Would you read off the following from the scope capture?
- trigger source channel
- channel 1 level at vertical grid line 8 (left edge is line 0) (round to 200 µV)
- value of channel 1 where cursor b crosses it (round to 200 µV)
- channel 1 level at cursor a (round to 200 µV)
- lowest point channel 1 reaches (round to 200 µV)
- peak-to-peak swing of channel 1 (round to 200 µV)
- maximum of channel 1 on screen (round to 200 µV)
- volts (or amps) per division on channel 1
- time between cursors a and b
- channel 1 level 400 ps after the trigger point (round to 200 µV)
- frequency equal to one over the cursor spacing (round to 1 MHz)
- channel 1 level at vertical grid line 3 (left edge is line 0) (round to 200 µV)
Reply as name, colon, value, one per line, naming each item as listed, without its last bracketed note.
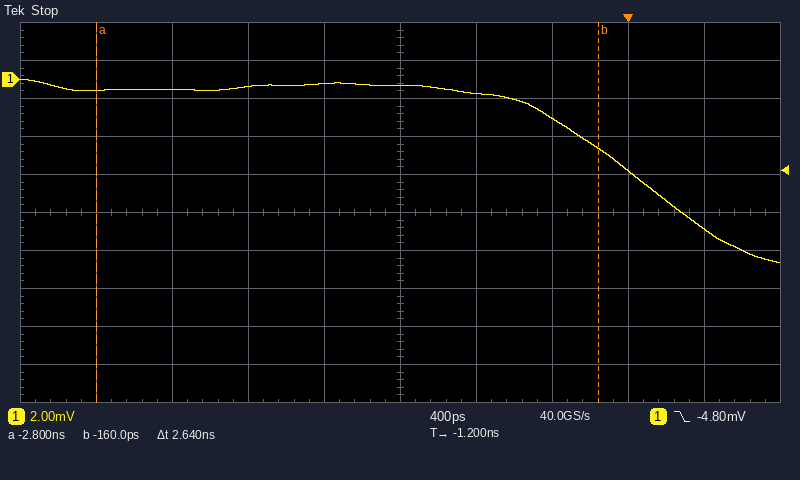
trigger source channel: channel 1
channel 1 level at vertical grid line 8 (left edge is line 0): -4.8 mV
value of channel 1 where cursor b crosses it: -3.6 mV
channel 1 level at cursor a: -600 µV
lowest point channel 1 reaches: -9.6 mV
peak-to-peak swing of channel 1: 9.6 mV
maximum of channel 1 on screen: 0.0 mV
volts (or amps) per division on channel 1: 2 mV
time between cursors a and b: 2.64 ns
channel 1 level 400 ps after the trigger point: -7.8 mV
frequency equal to one over the cursor spacing: 379 MHz
channel 1 level at vertical grid line 3 (left edge is line 0): -400 µV
